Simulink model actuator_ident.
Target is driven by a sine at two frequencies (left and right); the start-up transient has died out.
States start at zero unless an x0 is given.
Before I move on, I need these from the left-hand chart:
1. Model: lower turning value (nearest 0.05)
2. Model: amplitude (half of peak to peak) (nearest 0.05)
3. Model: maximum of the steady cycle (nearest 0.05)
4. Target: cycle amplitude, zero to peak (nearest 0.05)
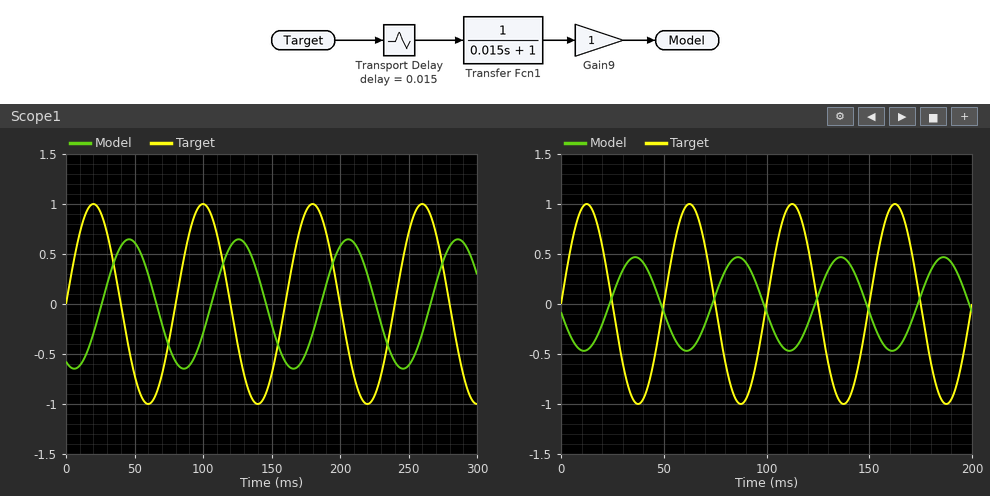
-0.65
0.65
0.65
1.00
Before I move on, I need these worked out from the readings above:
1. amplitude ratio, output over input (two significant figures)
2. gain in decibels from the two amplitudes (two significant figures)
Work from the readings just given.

0.65
-3.7 dB
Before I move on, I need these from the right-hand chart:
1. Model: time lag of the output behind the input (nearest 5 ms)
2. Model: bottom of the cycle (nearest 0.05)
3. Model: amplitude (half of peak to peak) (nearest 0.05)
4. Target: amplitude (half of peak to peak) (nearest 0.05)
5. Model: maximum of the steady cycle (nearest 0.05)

25 ms
-0.45
0.45
1.00
0.45
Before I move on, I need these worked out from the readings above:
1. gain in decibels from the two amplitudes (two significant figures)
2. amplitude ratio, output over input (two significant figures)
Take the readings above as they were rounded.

-6.9 dB
0.45
